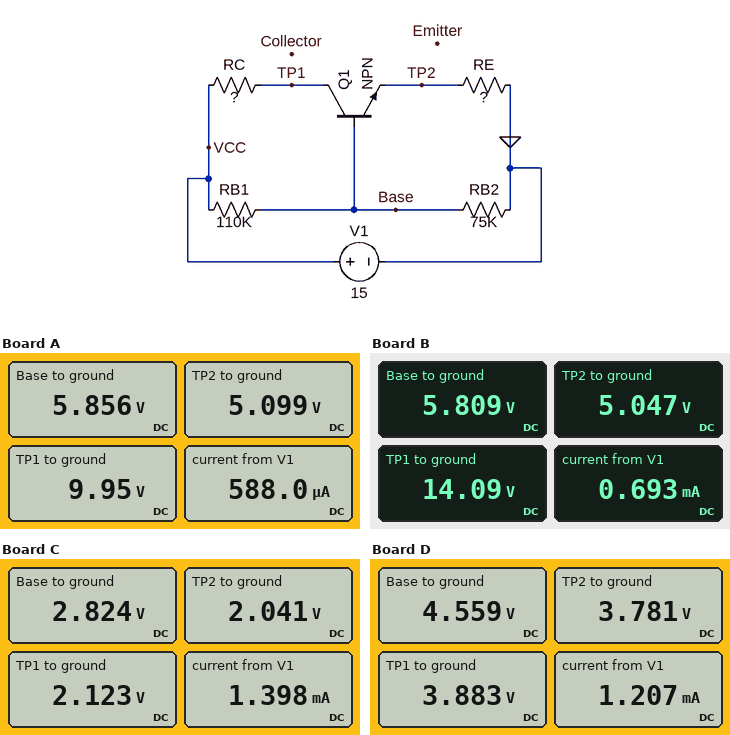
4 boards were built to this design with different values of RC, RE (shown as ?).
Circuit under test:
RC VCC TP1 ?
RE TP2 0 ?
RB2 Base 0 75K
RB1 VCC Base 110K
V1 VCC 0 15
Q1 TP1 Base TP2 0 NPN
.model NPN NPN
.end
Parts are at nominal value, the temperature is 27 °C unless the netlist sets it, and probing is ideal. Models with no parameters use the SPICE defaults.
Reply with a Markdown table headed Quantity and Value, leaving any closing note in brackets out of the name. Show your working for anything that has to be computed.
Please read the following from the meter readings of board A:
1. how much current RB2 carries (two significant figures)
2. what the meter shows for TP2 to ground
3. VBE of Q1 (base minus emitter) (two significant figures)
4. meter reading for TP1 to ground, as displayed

| Quantity | Value |
|---|---|
| how much current RB2 carries | (5.856 V) / 75 kΩ = 78 µA |
| what the meter shows for TP2 to ground | 5.099 V |
| VBE of Q1 (base minus emitter) | 5.856 V - 5.099 V = 760 mV |
| meter reading for TP1 to ground, as displayed | 9.95 V |
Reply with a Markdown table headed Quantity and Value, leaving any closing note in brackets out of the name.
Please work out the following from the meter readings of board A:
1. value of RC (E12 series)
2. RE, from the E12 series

| Quantity | Value |
|---|---|
| value of RC | 10 kΩ |
| RE, from the E12 series | 10 kΩ |
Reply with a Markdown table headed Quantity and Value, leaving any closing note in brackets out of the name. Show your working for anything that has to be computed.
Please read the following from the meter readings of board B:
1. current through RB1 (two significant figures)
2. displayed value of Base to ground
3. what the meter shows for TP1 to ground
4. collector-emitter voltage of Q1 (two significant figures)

| Quantity | Value |
|---|---|
| current through RB1 | (15 V - 5.809 V) / 110 kΩ = 84 µA |
| displayed value of Base to ground | 5.809 V |
| what the meter shows for TP1 to ground | 14.09 V |
| collector-emitter voltage of Q1 | 14.09 V - 5.047 V = 9.0 V |
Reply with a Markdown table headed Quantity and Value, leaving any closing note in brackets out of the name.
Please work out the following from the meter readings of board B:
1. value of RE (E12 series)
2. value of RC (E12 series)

| Quantity | Value |
|---|---|
| value of RE | 8.2 kΩ |
| value of RC | 1.5 kΩ |
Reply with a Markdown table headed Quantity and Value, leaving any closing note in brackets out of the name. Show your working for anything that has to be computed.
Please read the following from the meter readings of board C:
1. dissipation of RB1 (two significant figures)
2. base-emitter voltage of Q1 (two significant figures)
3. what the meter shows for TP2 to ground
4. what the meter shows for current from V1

| Quantity | Value |
|---|---|
| dissipation of RB1 | (15 V - 2.824 V)^2 / 110 kΩ = 1.3 mW |
| base-emitter voltage of Q1 | 2.824 V - 2.041 V = 780 mV |
| what the meter shows for TP2 to ground | 2.041 V |
| what the meter shows for current from V1 | 1.398 mA |
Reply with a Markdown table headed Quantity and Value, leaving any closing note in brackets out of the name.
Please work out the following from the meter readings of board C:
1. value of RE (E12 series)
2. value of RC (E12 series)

| Quantity | Value |
|---|---|
| value of RE | 1.5 kΩ |
| value of RC | 10 kΩ |
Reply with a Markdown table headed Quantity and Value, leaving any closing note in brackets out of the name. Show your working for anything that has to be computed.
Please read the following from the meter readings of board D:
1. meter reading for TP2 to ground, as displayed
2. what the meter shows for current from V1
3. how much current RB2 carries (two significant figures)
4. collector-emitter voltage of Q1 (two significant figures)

| Quantity | Value |
|---|---|
| meter reading for TP2 to ground, as displayed | 3.781 V |
| what the meter shows for current from V1 | 1.207 mA |
| how much current RB2 carries | (4.559 V) / 75 kΩ = 61 µA |
| collector-emitter voltage of Q1 | 3.883 V - 3.781 V = 100 mV |
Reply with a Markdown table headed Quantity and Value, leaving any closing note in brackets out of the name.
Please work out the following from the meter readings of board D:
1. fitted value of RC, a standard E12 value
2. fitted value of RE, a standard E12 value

| Quantity | Value |
|---|---|
| fitted value of RC, a standard E12 value | 10 kΩ |
| fitted value of RE, a standard E12 value | 3.3 kΩ |
